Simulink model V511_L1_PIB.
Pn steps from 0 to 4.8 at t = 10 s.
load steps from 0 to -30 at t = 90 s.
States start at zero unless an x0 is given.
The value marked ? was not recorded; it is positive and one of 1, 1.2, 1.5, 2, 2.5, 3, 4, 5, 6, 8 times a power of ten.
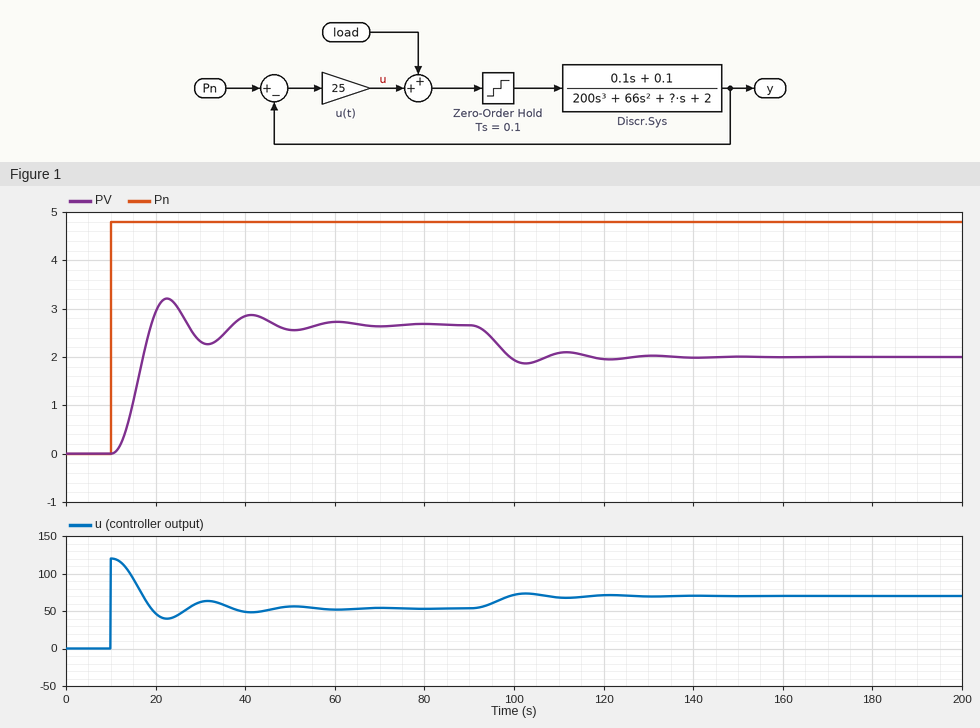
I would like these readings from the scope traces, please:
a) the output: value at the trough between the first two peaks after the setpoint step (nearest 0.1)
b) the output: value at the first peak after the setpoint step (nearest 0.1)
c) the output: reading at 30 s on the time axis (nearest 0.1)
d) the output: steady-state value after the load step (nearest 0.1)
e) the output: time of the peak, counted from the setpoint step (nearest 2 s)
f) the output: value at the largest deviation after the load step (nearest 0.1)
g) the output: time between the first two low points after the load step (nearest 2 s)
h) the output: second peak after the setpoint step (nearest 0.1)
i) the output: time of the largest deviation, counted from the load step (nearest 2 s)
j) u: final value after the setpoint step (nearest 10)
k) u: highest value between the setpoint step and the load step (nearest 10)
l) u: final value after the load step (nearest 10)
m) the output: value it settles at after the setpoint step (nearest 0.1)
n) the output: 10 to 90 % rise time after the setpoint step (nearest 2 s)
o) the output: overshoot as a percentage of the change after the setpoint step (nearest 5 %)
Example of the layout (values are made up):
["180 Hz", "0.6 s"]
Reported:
["2.3", "3.2", "2.3", "2.0", "12 s", "1.9", "18 s", "2.9", "12 s", "50", "120", "70", "2.7", "6 s", "20 %"]
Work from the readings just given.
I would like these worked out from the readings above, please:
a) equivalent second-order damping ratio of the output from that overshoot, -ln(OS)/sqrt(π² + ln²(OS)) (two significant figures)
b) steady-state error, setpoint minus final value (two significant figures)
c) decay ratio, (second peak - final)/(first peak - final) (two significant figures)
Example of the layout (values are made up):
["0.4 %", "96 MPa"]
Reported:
["0.46", "2.1", "0.40"]
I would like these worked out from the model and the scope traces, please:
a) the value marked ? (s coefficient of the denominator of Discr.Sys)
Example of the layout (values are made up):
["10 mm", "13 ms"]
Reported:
["25"]
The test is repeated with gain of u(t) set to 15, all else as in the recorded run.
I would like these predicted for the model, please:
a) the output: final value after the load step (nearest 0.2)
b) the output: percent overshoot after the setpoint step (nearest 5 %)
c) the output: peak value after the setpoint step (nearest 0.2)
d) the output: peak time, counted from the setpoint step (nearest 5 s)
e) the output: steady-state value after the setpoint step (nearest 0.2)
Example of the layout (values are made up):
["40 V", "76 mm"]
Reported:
["1.2", "10 %", "2.2", "15 s", "2.0"]
